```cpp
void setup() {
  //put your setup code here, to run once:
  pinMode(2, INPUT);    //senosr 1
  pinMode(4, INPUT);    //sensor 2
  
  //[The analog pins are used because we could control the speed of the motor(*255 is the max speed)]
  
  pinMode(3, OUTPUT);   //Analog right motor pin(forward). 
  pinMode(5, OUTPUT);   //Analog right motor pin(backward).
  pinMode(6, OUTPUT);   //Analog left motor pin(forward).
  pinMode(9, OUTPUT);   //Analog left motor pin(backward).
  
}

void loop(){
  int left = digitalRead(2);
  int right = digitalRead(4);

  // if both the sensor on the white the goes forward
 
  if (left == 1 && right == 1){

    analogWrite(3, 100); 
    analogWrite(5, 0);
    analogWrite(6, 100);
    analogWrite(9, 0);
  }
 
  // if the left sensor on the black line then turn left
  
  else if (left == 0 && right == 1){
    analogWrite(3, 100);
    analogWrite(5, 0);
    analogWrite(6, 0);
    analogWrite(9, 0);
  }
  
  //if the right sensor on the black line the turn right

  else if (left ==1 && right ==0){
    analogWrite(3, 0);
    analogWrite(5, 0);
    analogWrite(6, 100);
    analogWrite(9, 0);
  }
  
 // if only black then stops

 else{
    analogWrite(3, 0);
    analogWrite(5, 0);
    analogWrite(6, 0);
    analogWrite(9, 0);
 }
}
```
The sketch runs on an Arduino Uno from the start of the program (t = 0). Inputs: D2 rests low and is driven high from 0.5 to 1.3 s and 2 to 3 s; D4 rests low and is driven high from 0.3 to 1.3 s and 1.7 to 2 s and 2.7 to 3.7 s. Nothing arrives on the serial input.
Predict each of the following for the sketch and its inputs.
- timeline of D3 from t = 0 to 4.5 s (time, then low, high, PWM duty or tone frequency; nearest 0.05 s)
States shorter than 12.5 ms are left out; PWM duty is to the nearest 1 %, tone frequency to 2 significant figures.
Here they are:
0 s low; 0.3 s PWM 39 %; 1.3 s low; 1.7 s PWM 39 %; 2 s low; 2.7 s PWM 39 %; 3.7 s low
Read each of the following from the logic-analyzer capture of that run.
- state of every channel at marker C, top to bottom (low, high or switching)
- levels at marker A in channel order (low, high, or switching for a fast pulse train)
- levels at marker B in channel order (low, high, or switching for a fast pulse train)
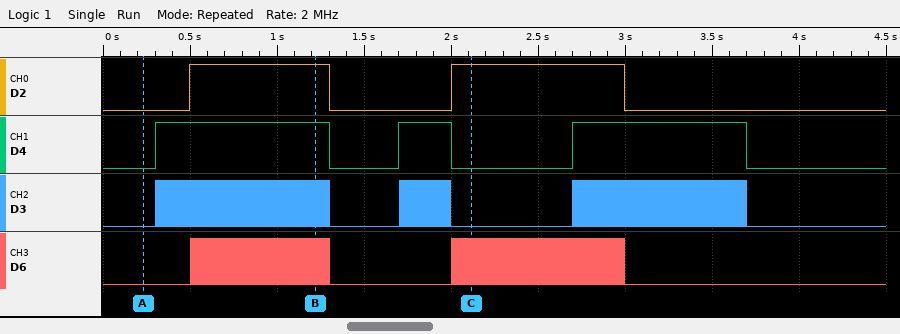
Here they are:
D2 high, D4 low, D3 low, D6 switching
D2 low, D4 low, D3 low, D6 low
D2 high, D4 high, D3 switching, D6 switching
